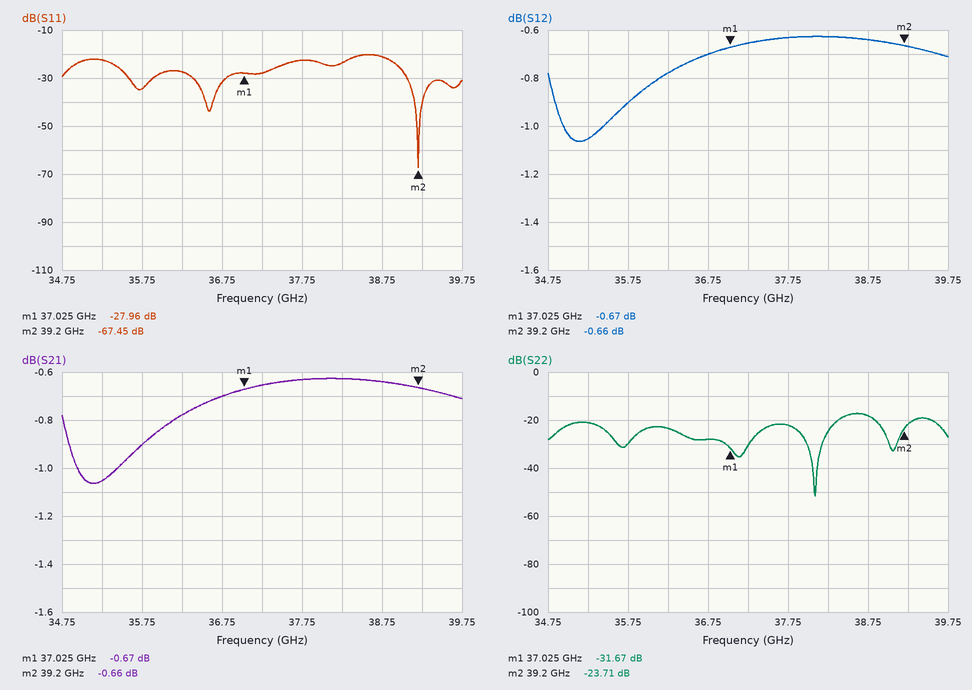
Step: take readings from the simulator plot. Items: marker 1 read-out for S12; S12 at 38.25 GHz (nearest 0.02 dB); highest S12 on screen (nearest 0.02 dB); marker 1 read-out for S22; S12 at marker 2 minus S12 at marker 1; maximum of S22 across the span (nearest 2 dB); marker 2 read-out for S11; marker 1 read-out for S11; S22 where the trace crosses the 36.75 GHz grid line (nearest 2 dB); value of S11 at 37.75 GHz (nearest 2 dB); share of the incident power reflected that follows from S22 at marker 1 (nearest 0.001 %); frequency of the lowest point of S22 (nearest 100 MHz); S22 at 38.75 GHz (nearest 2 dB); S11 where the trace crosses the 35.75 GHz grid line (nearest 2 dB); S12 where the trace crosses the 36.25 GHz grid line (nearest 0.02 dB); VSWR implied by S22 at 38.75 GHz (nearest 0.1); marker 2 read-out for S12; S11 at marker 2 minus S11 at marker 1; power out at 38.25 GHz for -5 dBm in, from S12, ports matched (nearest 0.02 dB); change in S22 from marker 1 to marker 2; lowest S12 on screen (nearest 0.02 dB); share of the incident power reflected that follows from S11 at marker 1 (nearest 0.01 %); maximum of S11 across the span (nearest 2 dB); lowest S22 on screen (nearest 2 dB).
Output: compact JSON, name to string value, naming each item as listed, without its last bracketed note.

{"marker 1 read-out for S12": "-0.67 dB", "S12 at 38.25 GHz": "-0.62 dB", "highest S12 on screen": "-0.62 dB", "marker 1 read-out for S22": "-31.67 dB", "S12 at marker 2 minus S12 at marker 1": "0.01 dB", "maximum of S22 across the span": "-18 dB", "marker 2 read-out for S11": "-67.45 dB", "marker 1 read-out for S11": "-27.96 dB", "S22 where the trace crosses the 36.75 GHz grid line": "-28 dB", "value of S11 at 37.75 GHz": "-22 dB", "share of the incident power reflected that follows from S22 at marker 1": "0.068 %", "frequency of the lowest point of S22": "38.1 GHz", "S22 at 38.75 GHz": "-18 dB", "S11 where the trace crosses the 35.75 GHz grid line": "-34 dB", "S12 where the trace crosses the 36.25 GHz grid line": "-0.78 dB", "VSWR implied by S22 at 38.75 GHz": "1.3", "marker 2 read-out for S12": "-0.66 dB", "S11 at marker 2 minus S11 at marker 1": "-39.49 dB", "power out at 38.25 GHz for -5 dBm in, from S12, ports matched": "-5.62 dBm", "change in S22 from marker 1 to marker 2": "7.96 dB", "lowest S12 on screen": "-1.06 dB", "share of the incident power reflected that follows from S11 at marker 1": "0.16 %", "maximum of S11 across the span": "-20 dB", "lowest S22 on screen": "-52 dB"}
